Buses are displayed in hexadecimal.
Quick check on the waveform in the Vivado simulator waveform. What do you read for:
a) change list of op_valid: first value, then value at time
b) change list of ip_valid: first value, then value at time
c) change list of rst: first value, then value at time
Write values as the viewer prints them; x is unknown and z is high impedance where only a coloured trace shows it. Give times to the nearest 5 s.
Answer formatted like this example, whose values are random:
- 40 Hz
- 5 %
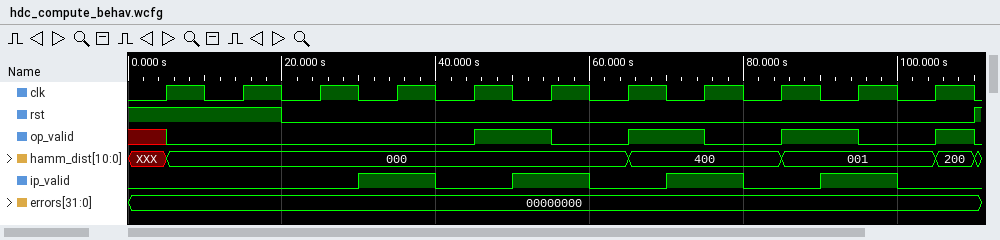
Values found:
- x, 0 at 5 s, 1 at 45 s, 0 at 55 s, 1 at 65 s, 0 at 75 s, 1 at 85 s, 0 at 95 s, 1 at 105 s, 0 at 110 s
- 0, 1 at 30 s, 0 at 40 s, 1 at 50 s, 0 at 60 s, 1 at 70 s, 0 at 80 s, 1 at 90 s, 0 at 100 s
- 1, 0 at 20 s, 1 at 110 s
